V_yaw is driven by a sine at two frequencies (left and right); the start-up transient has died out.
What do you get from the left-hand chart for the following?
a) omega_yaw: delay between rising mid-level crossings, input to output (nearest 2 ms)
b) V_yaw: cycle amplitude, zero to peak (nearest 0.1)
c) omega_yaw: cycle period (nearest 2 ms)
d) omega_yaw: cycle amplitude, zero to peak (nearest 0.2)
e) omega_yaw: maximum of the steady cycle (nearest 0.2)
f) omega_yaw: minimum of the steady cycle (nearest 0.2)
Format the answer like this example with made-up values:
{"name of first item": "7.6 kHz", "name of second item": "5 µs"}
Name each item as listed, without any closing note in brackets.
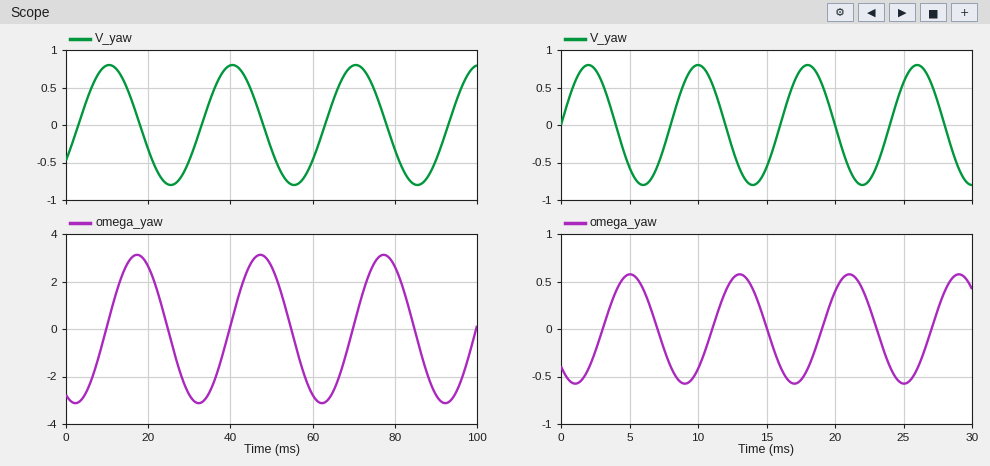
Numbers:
{"omega_yaw: delay between rising mid-level crossings, input to output": "6 ms", "V_yaw: cycle amplitude, zero to peak": "0.8", "omega_yaw: cycle period": "30 ms", "omega_yaw: cycle amplitude, zero to peak": "3.2", "omega_yaw: maximum of the steady cycle": "3.2", "omega_yaw: minimum of the steady cycle": "-3.2"}
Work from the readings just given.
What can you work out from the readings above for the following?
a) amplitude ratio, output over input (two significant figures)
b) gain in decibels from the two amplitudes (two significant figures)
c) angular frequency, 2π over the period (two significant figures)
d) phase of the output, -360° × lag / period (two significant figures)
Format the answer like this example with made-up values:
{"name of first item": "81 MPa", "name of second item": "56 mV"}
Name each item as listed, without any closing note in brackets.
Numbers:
{"amplitude ratio, output over input": "4.0", "gain in decibels from the two amplitudes": "12 dB", "angular frequency, 2π over the period": "0.21 rad/ms", "phase of the output, -360° × lag / period": "-72°"}
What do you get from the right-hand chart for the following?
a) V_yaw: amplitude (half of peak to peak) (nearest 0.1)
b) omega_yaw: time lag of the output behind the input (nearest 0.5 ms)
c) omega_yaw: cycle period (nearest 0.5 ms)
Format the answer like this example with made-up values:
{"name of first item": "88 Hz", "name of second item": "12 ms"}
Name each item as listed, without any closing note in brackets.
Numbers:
{"V_yaw: amplitude (half of peak to peak)": "0.8", "omega_yaw: time lag of the output behind the input": "3.0 ms", "omega_yaw: cycle period": "8.0 ms"}
